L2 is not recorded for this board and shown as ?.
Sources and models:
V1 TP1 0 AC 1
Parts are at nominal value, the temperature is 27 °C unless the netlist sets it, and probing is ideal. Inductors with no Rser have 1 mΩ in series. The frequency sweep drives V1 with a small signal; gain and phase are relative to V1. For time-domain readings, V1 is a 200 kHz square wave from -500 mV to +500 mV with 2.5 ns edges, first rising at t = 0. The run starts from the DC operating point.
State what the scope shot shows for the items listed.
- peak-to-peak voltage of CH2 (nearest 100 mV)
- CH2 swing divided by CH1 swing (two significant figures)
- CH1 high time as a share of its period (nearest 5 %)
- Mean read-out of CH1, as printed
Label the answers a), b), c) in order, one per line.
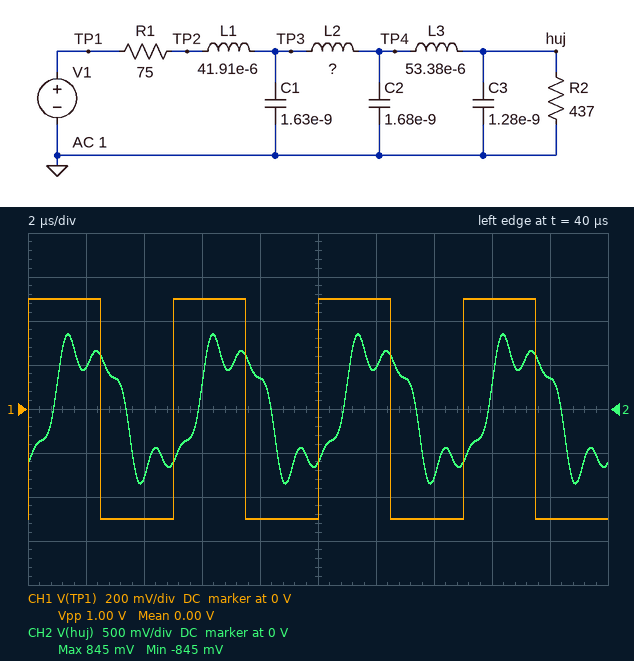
a) 1.7 V
b) 1.7
c) 50 %
d) 0.00 V
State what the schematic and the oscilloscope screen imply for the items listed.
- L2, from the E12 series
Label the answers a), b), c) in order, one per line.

a) 47 µH
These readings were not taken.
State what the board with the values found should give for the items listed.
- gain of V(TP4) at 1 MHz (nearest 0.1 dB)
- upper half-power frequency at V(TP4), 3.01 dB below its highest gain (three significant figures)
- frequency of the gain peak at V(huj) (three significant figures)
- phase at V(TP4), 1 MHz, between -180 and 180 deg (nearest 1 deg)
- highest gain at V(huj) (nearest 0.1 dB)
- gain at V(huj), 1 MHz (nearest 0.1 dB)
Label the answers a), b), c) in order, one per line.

a) 6.6 dB
b) 1.05 MHz
c) 267 kHz
d) 137 deg
e) 1.6 dB
f) 1.2 dB
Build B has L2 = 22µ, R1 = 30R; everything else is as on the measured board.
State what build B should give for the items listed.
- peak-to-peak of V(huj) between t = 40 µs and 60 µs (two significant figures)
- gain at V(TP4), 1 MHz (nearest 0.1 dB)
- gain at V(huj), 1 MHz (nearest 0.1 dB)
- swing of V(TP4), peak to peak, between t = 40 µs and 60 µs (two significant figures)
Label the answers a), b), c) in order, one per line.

a) 2.0 V
b) -5.6 dB
c) -11.0 dB
d) 1.6 V
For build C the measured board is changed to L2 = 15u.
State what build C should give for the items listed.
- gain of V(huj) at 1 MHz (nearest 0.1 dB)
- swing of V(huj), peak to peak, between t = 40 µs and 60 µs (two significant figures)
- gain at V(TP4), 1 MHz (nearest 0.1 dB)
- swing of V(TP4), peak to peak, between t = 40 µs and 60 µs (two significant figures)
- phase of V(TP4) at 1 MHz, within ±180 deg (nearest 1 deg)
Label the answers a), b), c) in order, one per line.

a) -13.3 dB
b) 1.4 V
c) -7.9 dB
d) 1.2 V
e) -160 deg
